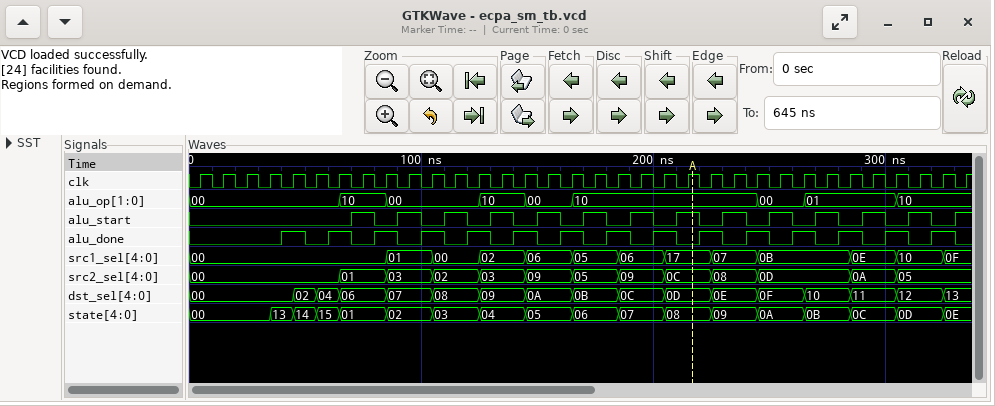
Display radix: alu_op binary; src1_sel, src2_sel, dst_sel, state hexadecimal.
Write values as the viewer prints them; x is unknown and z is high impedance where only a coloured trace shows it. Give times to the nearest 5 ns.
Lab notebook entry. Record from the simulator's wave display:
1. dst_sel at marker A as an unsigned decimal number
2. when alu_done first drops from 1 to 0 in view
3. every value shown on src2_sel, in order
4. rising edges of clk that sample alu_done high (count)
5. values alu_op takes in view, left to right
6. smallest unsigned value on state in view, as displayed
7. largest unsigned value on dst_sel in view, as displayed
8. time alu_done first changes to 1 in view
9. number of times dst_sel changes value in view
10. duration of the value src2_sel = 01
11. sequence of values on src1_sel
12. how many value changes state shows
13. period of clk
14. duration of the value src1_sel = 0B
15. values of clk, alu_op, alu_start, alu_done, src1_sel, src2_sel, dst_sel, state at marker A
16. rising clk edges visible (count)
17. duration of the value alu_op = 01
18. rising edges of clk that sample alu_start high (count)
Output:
13
50 ns
00, 01, 03, 02, 03, 09, 05, 09, 0C, 08, 0D, 0A, 05
15
00, 10, 00, 10, 00, 10, 00, 01, 10
00
13
40 ns
16
20 ns
00, 01, 00, 02, 06, 05, 06, 17, 07, 0B, 0E, 10, 0F
17
10 ns
40 ns
clk=1, alu_op=10, alu_start=1, alu_done=0, src1_sel=17, src2_sel=0C, dst_sel=0D, state=08
34
40 ns
14
